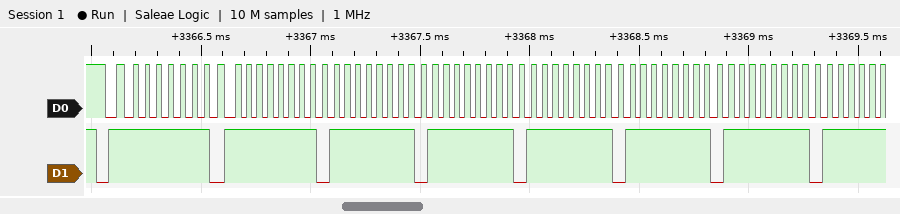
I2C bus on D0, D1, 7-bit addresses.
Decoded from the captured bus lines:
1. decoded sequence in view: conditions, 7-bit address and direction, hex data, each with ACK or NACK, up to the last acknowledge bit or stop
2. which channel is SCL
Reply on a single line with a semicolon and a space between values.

start, address 7F read ACK, FF ACK, FF ACK, FF ACK, FF ACK, FF ACK, FF ACK; D0
